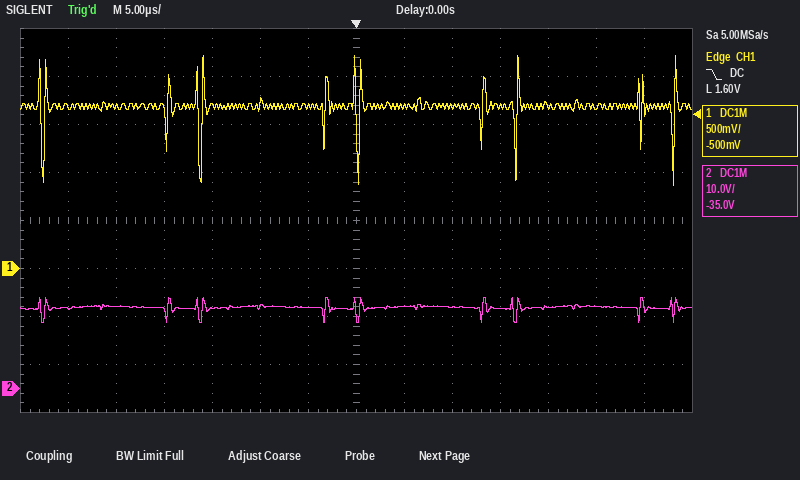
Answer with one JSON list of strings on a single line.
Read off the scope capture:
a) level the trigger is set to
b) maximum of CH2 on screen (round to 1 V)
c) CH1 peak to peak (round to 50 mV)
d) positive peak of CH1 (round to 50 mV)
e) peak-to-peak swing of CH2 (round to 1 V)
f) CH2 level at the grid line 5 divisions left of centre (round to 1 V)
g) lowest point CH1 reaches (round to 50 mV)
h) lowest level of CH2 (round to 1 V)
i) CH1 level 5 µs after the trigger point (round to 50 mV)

["1.60 V", "19 V", "1.35 V", "2.20 V", "5 V", "17 V", "850 mV", "14 V", "1.70 V"]
